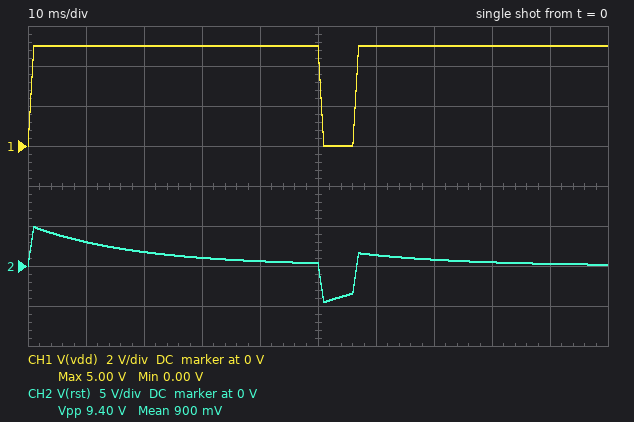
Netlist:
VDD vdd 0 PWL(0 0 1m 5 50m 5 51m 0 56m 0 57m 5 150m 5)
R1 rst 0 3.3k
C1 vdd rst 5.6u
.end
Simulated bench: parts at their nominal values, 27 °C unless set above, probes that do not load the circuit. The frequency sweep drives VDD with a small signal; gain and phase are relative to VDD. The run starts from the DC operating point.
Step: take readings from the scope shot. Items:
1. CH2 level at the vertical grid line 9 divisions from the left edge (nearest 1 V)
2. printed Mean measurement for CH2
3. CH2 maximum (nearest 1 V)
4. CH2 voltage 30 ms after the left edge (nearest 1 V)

0 V
900 mV
5 V
1 V
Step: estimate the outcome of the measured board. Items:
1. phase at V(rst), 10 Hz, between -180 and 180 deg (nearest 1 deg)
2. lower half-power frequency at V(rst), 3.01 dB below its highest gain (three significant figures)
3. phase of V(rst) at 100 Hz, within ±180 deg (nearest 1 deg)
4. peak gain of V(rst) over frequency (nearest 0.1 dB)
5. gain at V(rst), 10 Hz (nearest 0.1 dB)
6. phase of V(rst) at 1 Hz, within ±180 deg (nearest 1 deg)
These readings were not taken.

41 deg
8.61 Hz
5 deg
0 dB
-2.4 dB
83 deg
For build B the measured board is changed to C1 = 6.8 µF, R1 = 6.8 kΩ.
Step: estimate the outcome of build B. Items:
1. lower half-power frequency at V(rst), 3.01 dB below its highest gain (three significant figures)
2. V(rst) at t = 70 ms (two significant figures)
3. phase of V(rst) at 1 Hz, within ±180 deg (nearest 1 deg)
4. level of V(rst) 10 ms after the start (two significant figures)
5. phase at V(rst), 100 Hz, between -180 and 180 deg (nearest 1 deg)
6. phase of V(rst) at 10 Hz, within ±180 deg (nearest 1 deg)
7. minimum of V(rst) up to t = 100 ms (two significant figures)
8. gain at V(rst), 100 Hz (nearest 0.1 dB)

3.44 Hz
1.6 V
74 deg
4.1 V
2 deg
19 deg
-3.3 V
0 dB
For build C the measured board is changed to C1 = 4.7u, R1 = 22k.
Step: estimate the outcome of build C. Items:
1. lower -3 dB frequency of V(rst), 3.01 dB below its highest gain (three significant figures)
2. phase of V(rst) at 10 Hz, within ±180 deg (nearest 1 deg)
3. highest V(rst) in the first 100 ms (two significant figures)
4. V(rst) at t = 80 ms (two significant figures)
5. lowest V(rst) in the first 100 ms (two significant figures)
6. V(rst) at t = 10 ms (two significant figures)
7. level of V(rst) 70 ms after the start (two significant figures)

1.54 Hz
9 deg
5.0 V
2.5 V
-1.9 V
4.6 V
2.8 V
